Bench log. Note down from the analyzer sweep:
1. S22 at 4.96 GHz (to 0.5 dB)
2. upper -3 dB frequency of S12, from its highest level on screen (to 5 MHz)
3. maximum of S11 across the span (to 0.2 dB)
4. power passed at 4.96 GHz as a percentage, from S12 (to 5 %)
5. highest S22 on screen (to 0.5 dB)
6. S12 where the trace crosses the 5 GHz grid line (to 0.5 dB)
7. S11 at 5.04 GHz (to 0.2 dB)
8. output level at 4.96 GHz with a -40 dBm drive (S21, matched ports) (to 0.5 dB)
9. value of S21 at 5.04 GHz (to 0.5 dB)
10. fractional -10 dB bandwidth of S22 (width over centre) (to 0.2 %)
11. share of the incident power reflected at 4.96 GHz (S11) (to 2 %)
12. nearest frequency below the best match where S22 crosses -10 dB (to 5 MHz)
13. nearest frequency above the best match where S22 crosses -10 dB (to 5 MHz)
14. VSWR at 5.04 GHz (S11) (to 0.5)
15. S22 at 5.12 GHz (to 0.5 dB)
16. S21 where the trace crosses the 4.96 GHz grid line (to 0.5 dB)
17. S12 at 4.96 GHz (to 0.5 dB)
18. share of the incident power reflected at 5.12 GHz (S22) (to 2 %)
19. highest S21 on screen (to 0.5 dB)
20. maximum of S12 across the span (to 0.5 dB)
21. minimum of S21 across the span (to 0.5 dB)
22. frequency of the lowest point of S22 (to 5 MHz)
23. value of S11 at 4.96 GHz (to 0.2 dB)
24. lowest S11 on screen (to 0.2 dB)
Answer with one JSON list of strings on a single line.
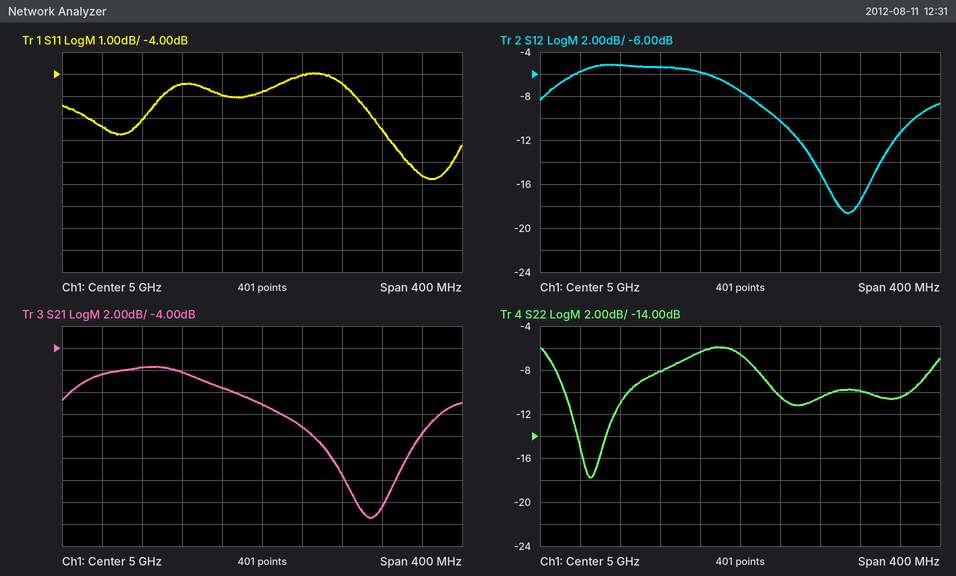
["-6.5 dB", "5.010 GHz", "-4.0 dB", "25 %", "-6.0 dB", "-7.5 dB", "-4.0 dB", "-47.5 dBm", "-11.0 dB", "1.4 %", "32 %", "4.825 GHz", "4.890 GHz", "4.5", "-10.0 dB", "-7.5 dB", "-6.0 dB", "10 %", "-5.5 dB", "-5.0 dB", "-19.5 dB", "4.850 GHz", "-5.0 dB", "-8.8 dB"]
